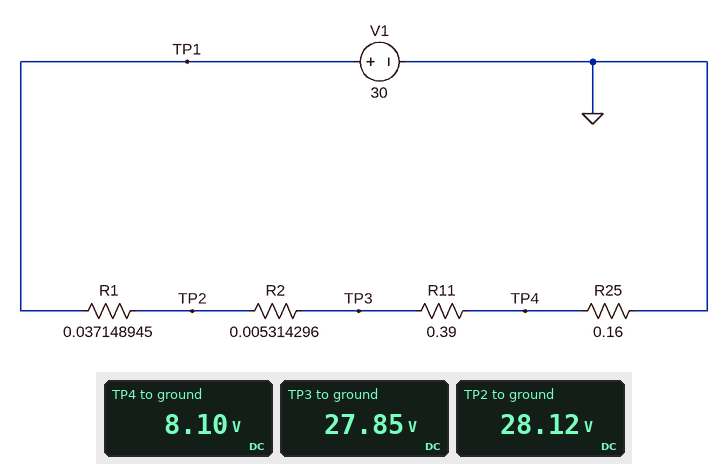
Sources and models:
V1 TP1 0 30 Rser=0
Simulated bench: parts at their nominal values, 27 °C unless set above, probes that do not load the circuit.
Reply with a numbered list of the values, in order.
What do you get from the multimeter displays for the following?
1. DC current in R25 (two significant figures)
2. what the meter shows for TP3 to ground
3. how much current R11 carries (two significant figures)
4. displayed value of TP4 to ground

1. 51 A
2. 27.85 V
3. 51 A
4. 8.10 V
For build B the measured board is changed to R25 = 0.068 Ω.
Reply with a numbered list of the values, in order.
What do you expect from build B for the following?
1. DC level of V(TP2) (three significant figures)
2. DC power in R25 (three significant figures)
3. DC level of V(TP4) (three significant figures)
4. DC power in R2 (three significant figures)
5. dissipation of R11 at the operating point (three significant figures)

1. 27.8 V
2. 244 W
3. 4.08 V
4. 19.1 W
5. 1.40 kW
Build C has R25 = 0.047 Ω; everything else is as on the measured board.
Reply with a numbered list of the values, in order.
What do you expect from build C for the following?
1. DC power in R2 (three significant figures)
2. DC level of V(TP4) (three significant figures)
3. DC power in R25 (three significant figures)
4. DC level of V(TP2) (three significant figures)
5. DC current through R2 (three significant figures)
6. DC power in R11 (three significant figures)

1. 20.8 W
2. 2.94 V
3. 184 W
4. 27.7 V
5. 62.6 A
6. 1.53 kW
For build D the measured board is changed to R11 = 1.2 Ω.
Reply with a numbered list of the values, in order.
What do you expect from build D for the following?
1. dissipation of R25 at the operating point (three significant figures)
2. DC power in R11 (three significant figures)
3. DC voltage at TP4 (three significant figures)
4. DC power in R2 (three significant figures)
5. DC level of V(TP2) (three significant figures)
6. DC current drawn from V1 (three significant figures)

1. 73.2 W
2. 549 W
3. 3.42 V
4. 2.43 W
5. 29.2 V
6. 21.4 A
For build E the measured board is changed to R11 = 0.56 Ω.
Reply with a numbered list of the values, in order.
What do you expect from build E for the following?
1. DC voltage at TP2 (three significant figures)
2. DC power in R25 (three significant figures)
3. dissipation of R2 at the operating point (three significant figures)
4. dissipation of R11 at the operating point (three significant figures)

1. 28.5 V
2. 248 W
3. 8.23 W
4. 867 W
